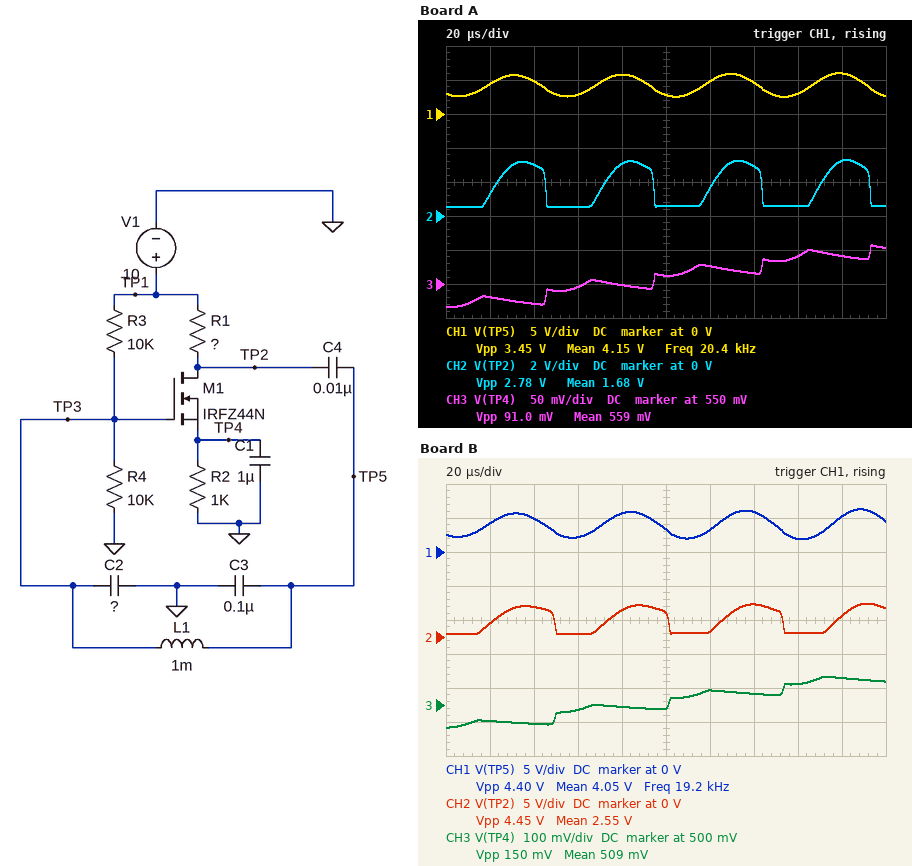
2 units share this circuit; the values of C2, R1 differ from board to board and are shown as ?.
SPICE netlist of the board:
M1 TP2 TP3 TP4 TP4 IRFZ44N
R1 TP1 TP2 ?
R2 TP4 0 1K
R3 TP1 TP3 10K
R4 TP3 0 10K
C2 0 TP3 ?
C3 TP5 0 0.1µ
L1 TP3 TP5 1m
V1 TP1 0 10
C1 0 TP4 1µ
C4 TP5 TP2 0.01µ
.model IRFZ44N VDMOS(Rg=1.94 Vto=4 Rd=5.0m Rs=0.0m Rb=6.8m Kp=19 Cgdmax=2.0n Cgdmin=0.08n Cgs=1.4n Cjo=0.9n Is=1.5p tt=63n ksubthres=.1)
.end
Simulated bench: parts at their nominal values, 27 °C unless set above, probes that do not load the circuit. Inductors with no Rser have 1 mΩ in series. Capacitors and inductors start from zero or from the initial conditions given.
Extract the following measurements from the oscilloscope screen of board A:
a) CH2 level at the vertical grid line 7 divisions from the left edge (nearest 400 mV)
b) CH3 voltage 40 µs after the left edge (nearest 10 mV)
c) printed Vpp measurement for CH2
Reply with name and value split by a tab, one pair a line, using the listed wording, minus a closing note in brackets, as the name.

CH2 level at the vertical grid line 7 divisions from the left edge	2.8 V
CH3 voltage 40 µs after the left edge	520 mV
printed Vpp measurement for CH2	2.78 V
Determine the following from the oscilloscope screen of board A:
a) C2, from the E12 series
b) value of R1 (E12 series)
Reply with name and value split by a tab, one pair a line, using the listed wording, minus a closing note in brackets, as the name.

C2, from the E12 series	150 nF
value of R1	8.2 kΩ
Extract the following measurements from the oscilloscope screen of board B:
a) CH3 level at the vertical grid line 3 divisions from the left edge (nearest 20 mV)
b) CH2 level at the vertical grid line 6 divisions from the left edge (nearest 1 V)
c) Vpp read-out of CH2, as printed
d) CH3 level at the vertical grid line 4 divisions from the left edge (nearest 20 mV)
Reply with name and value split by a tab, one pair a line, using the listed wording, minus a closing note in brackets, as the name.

CH3 level at the vertical grid line 3 divisions from the left edge	480 mV
CH2 level at the vertical grid line 6 divisions from the left edge	1 V
Vpp read-out of CH2, as printed	4.45 V
CH3 level at the vertical grid line 4 divisions from the left edge	500 mV
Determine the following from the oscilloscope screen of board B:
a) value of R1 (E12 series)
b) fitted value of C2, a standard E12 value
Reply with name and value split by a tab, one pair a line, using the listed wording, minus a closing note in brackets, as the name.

value of R1	5.6 kΩ
fitted value of C2, a standard E12 value	220 nF
